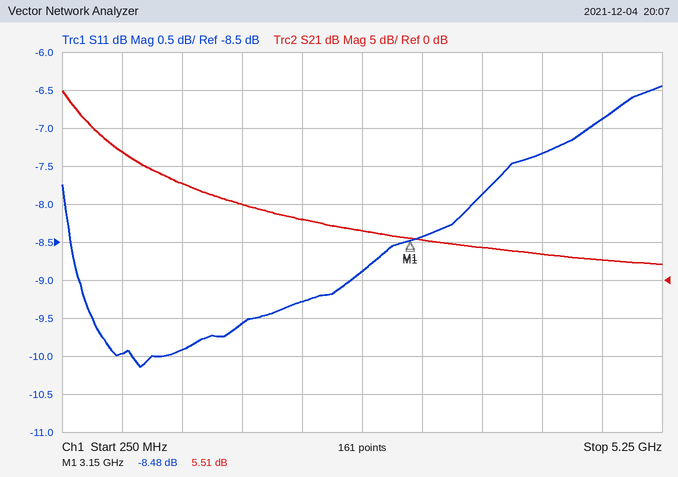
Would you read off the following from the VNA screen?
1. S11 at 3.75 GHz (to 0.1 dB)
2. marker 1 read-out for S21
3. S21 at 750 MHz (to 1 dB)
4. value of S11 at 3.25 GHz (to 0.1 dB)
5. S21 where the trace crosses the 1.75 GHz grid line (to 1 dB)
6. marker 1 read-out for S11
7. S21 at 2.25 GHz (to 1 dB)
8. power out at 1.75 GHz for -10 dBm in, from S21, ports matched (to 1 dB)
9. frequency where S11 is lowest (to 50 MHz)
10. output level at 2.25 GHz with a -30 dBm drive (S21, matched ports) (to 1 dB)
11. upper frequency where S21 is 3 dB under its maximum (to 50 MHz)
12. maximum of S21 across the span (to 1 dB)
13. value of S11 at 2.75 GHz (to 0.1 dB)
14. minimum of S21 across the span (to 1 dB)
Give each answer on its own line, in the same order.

-7.9 dB
5.51 dB
17 dB
-8.4 dB
10 dB
-8.48 dB
8 dB
0 dBm
900 MHz
-22 dBm
400 MHz
25 dB
-8.9 dB
2 dB
